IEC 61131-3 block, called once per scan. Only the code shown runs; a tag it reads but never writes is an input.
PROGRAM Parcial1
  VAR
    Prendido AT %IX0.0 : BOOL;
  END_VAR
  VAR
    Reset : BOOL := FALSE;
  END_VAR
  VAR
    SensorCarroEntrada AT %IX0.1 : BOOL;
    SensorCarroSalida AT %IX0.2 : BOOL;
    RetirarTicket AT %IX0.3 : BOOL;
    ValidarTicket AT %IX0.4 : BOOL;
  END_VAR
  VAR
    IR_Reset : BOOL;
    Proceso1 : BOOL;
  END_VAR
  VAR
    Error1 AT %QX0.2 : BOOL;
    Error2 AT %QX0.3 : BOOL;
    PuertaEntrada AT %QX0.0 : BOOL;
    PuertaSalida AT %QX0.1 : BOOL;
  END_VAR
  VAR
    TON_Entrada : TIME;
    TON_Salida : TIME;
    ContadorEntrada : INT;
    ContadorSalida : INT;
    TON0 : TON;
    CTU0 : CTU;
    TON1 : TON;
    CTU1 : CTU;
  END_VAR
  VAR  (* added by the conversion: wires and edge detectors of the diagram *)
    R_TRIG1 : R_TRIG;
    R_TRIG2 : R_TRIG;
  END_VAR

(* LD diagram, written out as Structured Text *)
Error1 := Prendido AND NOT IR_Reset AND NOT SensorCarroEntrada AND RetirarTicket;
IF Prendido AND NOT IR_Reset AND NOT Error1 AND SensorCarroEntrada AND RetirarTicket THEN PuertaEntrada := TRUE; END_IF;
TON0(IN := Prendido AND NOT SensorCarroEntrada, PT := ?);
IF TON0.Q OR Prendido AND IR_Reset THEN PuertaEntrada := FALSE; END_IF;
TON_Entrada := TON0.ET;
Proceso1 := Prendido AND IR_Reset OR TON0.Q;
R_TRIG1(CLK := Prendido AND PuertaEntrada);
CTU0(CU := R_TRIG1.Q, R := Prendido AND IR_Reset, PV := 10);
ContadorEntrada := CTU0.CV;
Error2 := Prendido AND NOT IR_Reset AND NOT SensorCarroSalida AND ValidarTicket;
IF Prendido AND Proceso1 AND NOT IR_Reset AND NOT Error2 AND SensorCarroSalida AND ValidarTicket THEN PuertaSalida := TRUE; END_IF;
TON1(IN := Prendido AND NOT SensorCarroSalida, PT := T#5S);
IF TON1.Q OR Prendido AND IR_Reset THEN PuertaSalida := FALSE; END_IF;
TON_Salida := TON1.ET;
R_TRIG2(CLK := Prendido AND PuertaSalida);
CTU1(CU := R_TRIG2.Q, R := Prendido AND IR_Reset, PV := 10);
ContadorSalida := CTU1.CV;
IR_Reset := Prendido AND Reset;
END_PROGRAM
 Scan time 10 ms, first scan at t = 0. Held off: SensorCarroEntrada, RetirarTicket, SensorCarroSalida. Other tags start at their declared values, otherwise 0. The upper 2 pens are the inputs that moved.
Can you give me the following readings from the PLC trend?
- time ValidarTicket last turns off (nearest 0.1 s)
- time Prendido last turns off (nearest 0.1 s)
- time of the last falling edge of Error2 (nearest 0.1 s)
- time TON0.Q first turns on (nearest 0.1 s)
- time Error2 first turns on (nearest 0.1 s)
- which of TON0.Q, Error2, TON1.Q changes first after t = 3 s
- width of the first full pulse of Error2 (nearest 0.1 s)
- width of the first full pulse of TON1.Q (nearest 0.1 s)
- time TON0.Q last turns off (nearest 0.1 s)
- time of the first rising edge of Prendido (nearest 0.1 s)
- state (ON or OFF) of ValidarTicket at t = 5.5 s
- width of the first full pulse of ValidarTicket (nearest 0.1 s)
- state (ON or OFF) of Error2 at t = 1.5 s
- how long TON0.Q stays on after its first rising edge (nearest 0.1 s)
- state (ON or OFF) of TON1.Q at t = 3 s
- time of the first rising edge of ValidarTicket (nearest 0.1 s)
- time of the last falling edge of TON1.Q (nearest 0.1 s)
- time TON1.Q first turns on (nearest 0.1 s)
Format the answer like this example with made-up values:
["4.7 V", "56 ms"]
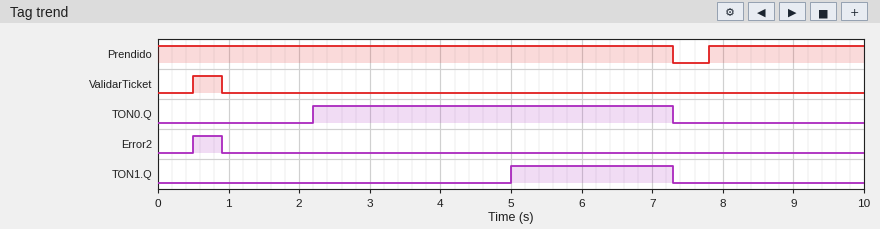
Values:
["0.9 s", "7.3 s", "0.9 s", "2.2 s", "0.5 s", "TON1.Q", "0.4 s", "2.3 s", "7.3 s", "7.8 s", "OFF", "0.4 s", "OFF", "5.1 s", "OFF", "0.5 s", "7.3 s", "5.0 s"]
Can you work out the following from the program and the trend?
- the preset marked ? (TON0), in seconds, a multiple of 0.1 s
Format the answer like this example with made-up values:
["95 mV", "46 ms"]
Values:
["2.2 s"]
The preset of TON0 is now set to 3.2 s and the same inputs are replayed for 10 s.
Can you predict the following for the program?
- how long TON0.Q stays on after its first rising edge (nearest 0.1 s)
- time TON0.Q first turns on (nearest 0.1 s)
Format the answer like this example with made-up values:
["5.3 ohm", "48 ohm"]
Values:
["4.1 s", "3.2 s"]
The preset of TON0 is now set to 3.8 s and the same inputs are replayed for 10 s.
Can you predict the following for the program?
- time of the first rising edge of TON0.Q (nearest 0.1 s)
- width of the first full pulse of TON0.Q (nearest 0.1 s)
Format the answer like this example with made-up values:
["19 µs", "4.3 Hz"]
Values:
["3.8 s", "3.5 s"]
